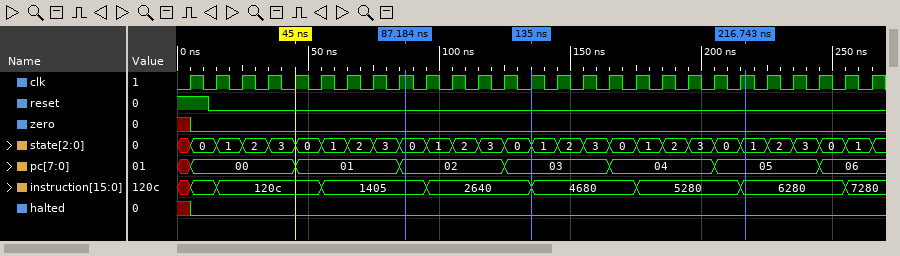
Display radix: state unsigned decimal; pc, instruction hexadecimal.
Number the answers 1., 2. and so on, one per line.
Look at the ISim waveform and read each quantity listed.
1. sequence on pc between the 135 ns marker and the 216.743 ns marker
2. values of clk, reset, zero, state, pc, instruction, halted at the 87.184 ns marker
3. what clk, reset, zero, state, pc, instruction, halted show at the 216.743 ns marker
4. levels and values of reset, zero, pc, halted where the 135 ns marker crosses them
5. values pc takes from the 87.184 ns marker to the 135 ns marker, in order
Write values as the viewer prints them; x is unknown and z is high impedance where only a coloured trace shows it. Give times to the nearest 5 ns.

1. 03, 04, 05
2. clk=1, reset=0, zero=0, state=0, pc=02, instruction=1405, halted=0
3. clk=1, reset=0, zero=0, state=1, pc=05, instruction=6280, halted=0
4. reset=0, zero=0, pc=03, halted=0
5. 02, 03
